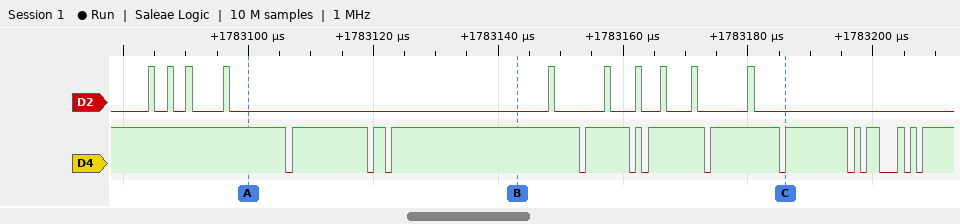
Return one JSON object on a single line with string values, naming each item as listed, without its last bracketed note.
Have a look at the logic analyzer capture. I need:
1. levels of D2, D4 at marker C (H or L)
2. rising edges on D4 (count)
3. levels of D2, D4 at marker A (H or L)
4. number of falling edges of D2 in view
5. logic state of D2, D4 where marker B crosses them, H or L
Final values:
{"levels of D2, D4 at marker C": "D2=L, D4=H", "rising edges on D4": "13", "levels of D2, D4 at marker A": "D2=L, D4=H", "number of falling edges of D2 in view": "10", "logic state of D2, D4 where marker B crosses them, H or L": "D2=L, D4=H"}
